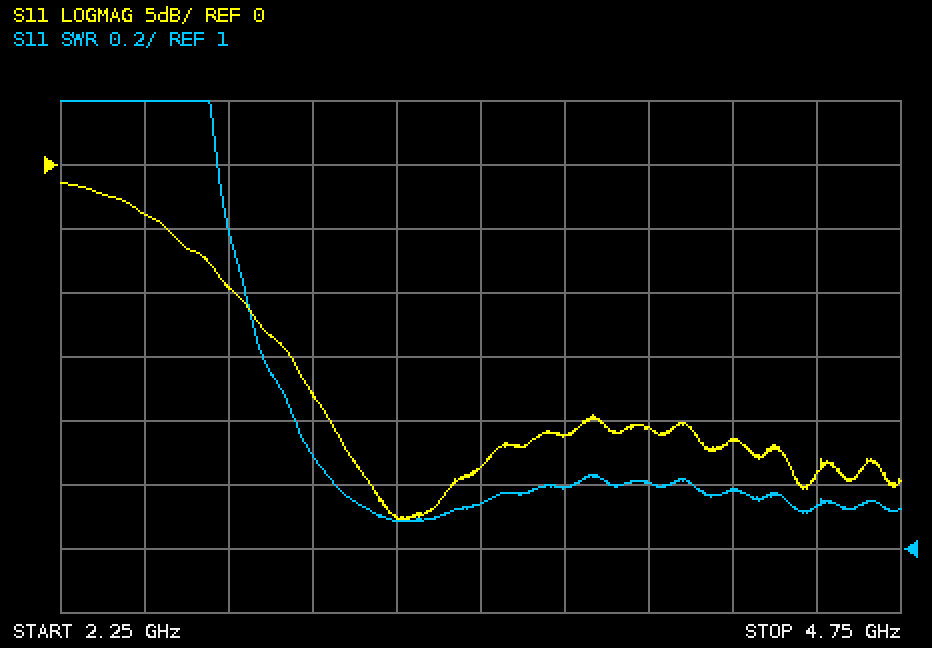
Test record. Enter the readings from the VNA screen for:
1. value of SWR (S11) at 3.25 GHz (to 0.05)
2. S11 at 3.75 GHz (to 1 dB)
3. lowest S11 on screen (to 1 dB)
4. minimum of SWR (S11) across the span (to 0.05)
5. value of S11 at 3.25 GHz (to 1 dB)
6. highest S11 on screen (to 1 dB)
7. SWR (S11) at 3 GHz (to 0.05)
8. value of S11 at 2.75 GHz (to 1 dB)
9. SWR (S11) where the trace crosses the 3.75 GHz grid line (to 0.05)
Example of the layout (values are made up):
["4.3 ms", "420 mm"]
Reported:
["1.10", "-21 dB", "-28 dB", "1.10", "-28 dB", "-1 dB", "1.30", "-10 dB", "1.20"]
